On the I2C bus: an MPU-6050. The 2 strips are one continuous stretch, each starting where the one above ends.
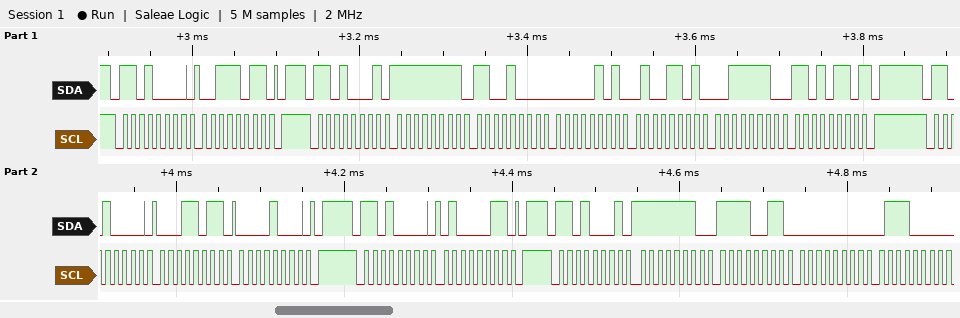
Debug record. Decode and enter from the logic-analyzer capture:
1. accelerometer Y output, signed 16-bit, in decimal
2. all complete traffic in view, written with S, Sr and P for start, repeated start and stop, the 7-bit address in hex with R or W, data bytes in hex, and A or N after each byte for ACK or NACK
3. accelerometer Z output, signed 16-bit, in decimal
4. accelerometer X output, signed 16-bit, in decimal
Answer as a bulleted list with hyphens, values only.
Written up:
- 1357
- S 68W A 3B A P S 68R A FF A C8 A 05 A 4D A 3E A D6 N P S 68W A 1B A 08 A P S 68W A 43 A P S 68R A FE A F3 A 00 A 70 A
- 16086
- -56
